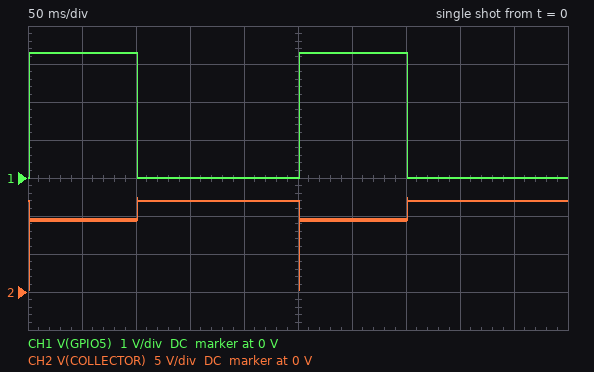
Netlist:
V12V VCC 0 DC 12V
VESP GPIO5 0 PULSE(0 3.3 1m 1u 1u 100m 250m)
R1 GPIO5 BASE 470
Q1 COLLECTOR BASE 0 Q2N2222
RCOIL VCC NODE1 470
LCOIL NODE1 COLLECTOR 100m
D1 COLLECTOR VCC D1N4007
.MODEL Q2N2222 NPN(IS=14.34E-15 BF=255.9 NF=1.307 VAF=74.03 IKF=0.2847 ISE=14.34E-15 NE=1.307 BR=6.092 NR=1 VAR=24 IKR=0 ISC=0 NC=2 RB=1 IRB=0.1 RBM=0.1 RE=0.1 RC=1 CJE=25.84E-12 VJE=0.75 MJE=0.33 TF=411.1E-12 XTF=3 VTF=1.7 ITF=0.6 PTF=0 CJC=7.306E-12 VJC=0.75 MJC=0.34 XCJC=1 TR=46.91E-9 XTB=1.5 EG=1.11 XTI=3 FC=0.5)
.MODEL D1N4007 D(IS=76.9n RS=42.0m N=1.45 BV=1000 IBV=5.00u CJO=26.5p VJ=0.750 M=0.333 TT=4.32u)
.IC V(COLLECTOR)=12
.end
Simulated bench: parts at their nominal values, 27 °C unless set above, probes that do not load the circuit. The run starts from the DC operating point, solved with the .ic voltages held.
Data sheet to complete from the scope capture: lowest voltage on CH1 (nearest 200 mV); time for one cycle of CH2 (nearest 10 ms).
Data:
0 V
250 ms
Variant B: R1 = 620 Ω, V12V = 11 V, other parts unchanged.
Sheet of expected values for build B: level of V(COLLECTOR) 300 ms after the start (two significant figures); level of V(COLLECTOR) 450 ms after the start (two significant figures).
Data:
9.1 V
11 V
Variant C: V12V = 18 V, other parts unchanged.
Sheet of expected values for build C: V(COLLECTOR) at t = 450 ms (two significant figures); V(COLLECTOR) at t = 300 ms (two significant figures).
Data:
18 V
15 V
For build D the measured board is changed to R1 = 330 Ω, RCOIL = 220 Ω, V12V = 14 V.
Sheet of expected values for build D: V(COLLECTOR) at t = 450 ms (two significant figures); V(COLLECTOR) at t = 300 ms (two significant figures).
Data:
14 V
12 V
